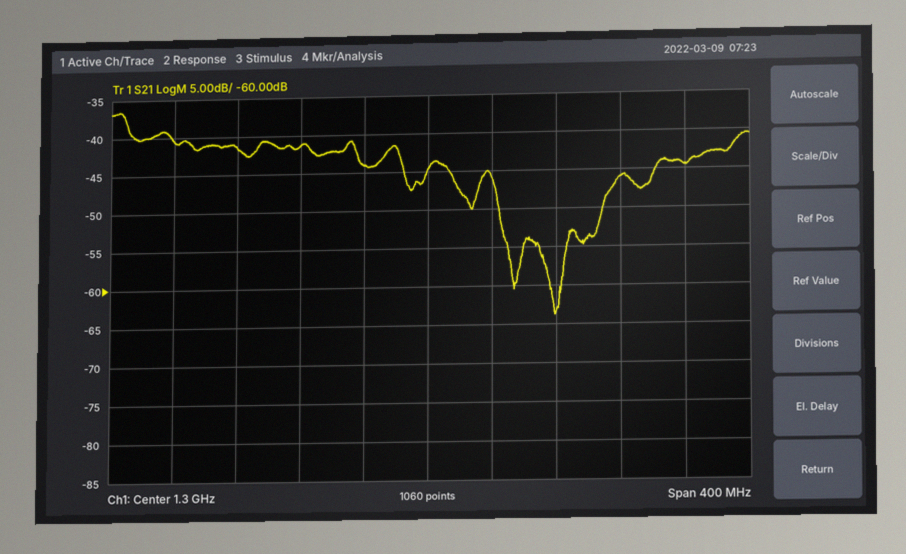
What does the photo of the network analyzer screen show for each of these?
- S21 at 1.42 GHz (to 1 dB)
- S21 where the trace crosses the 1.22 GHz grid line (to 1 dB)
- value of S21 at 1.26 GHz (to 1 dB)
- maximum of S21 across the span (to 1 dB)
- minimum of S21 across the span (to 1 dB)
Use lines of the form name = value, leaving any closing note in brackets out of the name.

S21 at 1.42 GHz = -46 dB
S21 where the trace crosses the 1.22 GHz grid line = -41 dB
value of S21 at 1.26 GHz = -44 dB
maximum of S21 across the span = -37 dB
minimum of S21 across the span = -64 dB
